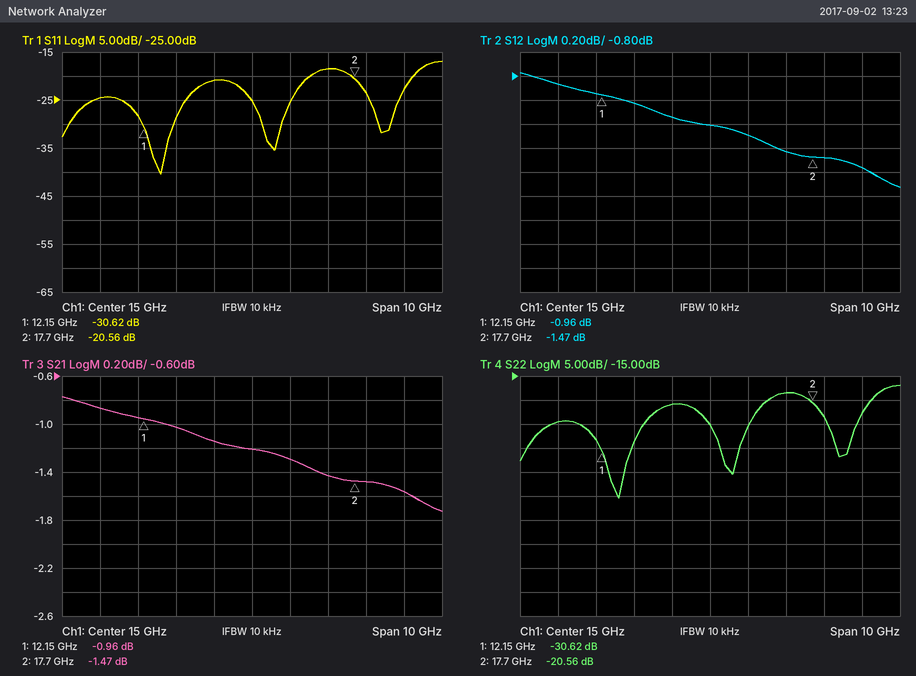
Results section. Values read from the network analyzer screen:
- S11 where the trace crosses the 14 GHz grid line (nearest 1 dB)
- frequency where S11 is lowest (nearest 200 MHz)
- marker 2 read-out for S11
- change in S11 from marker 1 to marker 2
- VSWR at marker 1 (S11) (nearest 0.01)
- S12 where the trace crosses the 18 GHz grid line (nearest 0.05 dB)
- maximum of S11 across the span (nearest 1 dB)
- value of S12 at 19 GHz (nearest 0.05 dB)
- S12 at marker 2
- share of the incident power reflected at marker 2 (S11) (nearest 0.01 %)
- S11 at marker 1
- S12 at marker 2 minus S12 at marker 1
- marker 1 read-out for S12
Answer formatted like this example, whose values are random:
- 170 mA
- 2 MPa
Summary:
- -21 dB
- 12.6 GHz
- -20.56 dB
- 10.06 dB
- 1.06
- -1.50 dB
- -17 dB
- -1.55 dB
- -1.47 dB
- 0.88 %
- -30.62 dB
- -0.51 dB
- -0.96 dB
